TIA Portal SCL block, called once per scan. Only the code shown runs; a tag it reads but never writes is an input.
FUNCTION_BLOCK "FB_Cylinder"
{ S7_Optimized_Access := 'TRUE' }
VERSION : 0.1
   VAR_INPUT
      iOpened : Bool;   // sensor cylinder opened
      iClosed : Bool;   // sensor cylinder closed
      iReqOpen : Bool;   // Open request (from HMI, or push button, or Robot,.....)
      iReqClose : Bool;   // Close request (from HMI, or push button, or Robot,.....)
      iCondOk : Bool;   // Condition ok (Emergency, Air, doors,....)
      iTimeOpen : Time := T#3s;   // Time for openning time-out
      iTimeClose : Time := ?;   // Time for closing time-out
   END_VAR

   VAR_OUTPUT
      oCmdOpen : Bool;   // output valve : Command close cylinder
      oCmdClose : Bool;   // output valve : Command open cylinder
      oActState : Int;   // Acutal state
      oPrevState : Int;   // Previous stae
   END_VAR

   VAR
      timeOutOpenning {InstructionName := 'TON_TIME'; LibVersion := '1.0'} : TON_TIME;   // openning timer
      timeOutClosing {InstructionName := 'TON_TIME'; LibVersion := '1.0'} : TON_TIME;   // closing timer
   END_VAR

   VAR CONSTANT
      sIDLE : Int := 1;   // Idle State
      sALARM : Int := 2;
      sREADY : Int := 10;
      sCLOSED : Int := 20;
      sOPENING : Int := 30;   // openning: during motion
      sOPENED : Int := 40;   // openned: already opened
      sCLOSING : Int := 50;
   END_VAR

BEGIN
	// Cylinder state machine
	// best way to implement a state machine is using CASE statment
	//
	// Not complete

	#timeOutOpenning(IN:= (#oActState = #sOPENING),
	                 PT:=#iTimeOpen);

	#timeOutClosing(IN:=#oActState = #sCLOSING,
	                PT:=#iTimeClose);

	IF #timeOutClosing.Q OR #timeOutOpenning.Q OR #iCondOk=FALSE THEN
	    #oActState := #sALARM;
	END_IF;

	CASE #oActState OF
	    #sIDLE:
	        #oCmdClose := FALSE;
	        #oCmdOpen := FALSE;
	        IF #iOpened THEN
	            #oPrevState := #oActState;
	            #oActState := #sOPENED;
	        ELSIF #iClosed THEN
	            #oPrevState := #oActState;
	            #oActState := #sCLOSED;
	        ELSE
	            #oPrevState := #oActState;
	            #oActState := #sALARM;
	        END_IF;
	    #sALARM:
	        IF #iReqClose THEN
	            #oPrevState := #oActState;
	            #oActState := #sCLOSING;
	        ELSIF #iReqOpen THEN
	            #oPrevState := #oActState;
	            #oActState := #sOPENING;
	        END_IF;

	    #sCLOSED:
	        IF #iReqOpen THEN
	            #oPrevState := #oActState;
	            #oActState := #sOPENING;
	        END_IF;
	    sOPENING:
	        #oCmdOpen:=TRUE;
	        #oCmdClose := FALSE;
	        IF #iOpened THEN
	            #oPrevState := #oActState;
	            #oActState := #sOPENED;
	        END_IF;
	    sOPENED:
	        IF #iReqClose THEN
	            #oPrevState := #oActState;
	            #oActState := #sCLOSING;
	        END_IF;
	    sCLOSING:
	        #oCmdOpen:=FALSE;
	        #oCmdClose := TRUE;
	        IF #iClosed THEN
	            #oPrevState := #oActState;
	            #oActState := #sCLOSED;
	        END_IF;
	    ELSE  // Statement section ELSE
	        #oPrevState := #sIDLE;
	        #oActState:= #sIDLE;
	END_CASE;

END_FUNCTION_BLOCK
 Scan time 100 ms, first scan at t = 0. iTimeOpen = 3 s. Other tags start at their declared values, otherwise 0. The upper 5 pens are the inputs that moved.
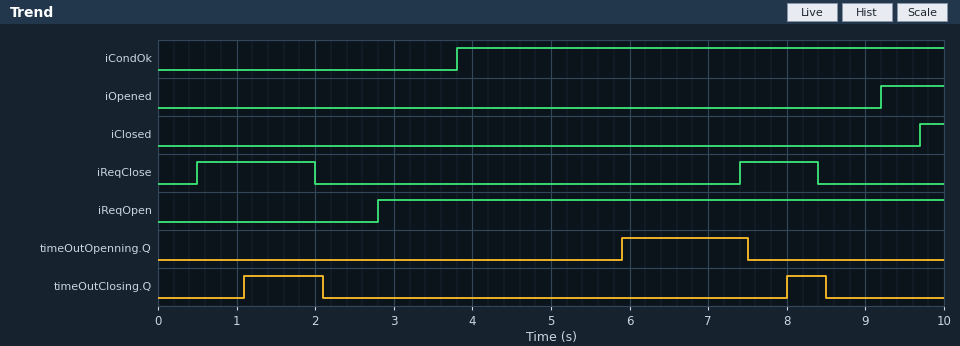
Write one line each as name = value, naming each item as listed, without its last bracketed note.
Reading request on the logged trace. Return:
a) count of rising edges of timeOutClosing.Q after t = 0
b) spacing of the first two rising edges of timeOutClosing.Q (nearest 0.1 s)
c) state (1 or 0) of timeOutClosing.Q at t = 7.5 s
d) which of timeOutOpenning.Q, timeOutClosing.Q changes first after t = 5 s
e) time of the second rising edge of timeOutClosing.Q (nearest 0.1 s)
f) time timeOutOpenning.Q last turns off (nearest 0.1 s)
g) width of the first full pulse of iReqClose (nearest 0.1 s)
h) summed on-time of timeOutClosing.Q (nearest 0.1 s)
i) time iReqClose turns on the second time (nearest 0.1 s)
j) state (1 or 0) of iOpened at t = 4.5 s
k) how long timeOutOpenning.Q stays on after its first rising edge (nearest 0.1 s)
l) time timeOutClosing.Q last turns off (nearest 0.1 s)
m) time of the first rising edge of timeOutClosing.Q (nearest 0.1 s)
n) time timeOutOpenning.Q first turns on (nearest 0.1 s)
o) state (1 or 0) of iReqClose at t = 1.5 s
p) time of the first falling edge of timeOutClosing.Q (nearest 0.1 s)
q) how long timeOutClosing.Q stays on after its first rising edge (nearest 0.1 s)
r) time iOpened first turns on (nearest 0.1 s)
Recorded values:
count of rising edges of timeOutClosing.Q after t = 0 = 2
spacing of the first two rising edges of timeOutClosing.Q = 6.9 s
state (1 or 0) of timeOutClosing.Q at t = 7.5 s = 0
which of timeOutOpenning.Q, timeOutClosing.Q changes first after t = 5 s = timeOutOpenning.Q
time of the second rising edge of timeOutClosing.Q = 8.0 s
time timeOutOpenning.Q last turns off = 7.5 s
width of the first full pulse of iReqClose = 1.5 s
summed on-time of timeOutClosing.Q = 1.5 s
time iReqClose turns on the second time = 7.4 s
state (1 or 0) of iOpened at t = 4.5 s = 0
how long timeOutOpenning.Q stays on after its first rising edge = 1.6 s
time timeOutClosing.Q last turns off = 8.5 s
time of the first rising edge of timeOutClosing.Q = 1.1 s
time timeOutOpenning.Q first turns on = 5.9 s
state (1 or 0) of iReqClose at t = 1.5 s = 1
time of the first falling edge of timeOutClosing.Q = 2.1 s
how long timeOutClosing.Q stays on after its first rising edge = 1.0 s
time iOpened first turns on = 9.2 s
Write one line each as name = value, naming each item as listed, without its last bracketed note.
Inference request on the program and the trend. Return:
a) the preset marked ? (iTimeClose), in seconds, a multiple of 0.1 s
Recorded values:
the preset marked ? (iTimeClose), in seconds, a multiple of 0.1 s = 0.5 s
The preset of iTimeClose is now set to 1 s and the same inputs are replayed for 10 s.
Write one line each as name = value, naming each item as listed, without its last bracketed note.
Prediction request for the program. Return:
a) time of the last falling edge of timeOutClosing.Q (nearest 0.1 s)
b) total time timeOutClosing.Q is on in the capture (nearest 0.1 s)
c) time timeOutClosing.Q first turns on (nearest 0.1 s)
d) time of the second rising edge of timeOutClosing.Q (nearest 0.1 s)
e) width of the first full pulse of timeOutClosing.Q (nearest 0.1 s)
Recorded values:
time of the last falling edge of timeOutClosing.Q = 8.6 s
total time timeOutClosing.Q is on in the capture = 0.6 s
time timeOutClosing.Q first turns on = 1.6 s
time of the second rising edge of timeOutClosing.Q = 8.5 s
width of the first full pulse of timeOutClosing.Q = 0.5 s
